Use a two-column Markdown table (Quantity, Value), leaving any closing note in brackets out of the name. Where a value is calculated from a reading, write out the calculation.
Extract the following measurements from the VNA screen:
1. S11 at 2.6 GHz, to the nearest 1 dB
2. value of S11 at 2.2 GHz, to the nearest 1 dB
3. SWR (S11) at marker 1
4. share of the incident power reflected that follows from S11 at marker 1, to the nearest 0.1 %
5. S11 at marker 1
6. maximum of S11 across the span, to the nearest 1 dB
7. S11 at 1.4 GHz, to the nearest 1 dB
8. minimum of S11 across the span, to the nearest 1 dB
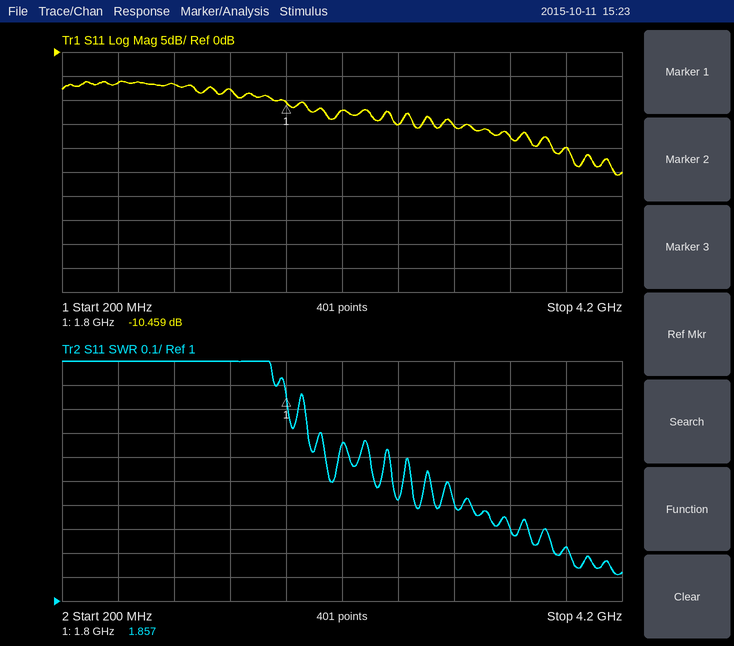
| Quantity | Value |
|---|---|
| S11 at 2.6 GHz, to the nearest 1 dB | -15 dB |
| value of S11 at 2.2 GHz, to the nearest 1 dB | -12 dB |
| SWR (S11) at marker 1 | 1.857 |
| share of the incident power reflected that follows from S11 at marker 1, to the nearest 0.1 % | 10^(-10.459/10) ≈ 9.0 % |
| S11 at marker 1 | -10.459 dB |
| maximum of S11 across the span, to the nearest 1 dB | -6 dB |
| S11 at 1.4 GHz, to the nearest 1 dB | -8 dB |
| minimum of S11 across the span, to the nearest 1 dB | -26 dB |
